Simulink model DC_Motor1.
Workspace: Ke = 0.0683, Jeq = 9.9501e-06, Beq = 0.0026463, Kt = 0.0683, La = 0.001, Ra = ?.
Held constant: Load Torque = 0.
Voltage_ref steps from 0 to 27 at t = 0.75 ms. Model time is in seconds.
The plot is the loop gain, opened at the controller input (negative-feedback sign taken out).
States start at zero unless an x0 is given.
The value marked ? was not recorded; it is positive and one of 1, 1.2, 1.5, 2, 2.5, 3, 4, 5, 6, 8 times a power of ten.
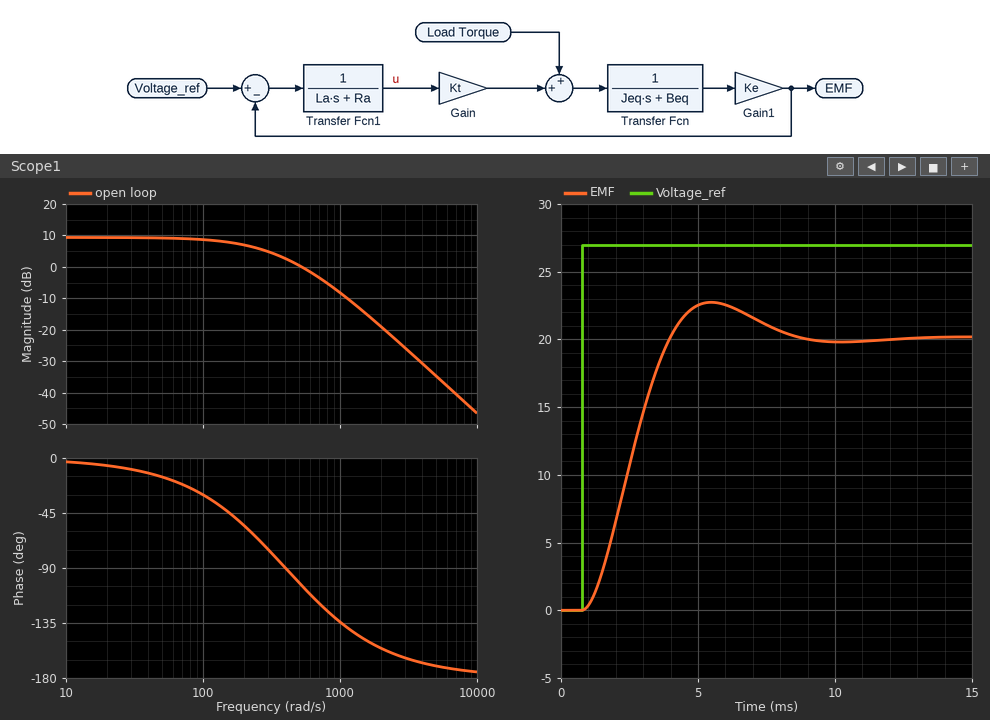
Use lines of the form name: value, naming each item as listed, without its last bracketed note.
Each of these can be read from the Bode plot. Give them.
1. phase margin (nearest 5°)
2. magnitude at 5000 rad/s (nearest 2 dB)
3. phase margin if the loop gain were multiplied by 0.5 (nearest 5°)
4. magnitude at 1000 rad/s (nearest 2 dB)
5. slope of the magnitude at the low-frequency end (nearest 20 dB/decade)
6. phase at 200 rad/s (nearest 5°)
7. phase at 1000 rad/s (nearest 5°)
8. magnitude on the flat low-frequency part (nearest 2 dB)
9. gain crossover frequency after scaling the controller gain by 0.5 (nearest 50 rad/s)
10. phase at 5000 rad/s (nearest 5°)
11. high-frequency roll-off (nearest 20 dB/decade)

phase margin: 75°
magnitude at 5000 rad/s: -34 dB
phase margin if the loop gain were multiplied by 0.5: 115°
magnitude at 1000 rad/s: -8 dB
slope of the magnitude at the low-frequency end: 0 dB/decade
phase at 200 rad/s: -55°
phase at 1000 rad/s: -135°
magnitude on the flat low-frequency part: 10 dB
gain crossover frequency after scaling the controller gain by 0.5: 250 rad/s
phase at 5000 rad/s: -170°
high-frequency roll-off: -40 dB/decade
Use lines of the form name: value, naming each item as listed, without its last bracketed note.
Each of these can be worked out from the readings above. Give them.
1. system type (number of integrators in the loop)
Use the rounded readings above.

system type: 0
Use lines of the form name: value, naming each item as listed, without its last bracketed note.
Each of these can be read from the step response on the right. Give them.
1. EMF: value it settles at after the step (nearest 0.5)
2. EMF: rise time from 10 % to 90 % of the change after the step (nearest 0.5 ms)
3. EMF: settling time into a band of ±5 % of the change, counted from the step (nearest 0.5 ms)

EMF: value it settles at after the step: 20.0
EMF: rise time from 10 % to 90 % of the change after the step: 2.0 ms
EMF: settling time into a band of ±5 % of the change, counted from the step: 6.5 ms
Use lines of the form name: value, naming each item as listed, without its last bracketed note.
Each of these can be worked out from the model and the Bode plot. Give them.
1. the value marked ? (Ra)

the value marked ?: 0.6
